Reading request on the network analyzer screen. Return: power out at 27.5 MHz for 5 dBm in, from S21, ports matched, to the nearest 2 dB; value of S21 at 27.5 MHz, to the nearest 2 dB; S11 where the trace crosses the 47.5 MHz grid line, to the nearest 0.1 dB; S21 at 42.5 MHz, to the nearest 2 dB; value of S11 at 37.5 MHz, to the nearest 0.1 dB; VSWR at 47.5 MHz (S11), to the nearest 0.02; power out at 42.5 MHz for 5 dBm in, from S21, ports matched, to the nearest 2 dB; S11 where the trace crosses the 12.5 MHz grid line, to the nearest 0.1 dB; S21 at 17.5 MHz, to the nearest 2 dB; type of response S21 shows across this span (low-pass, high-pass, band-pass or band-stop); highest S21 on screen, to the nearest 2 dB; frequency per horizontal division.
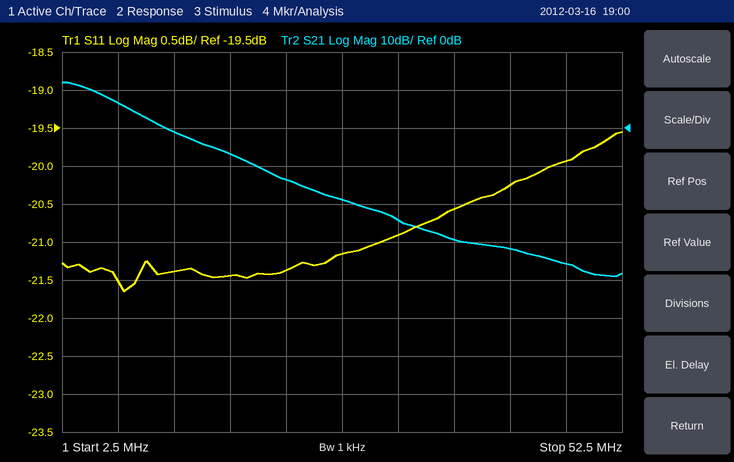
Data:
-14 dBm
-18 dB
-19.9 dB
-32 dB
-20.6 dB
1.22
-26 dBm
-21.4 dB
-6 dB
low-pass
12 dB
5 MHz
